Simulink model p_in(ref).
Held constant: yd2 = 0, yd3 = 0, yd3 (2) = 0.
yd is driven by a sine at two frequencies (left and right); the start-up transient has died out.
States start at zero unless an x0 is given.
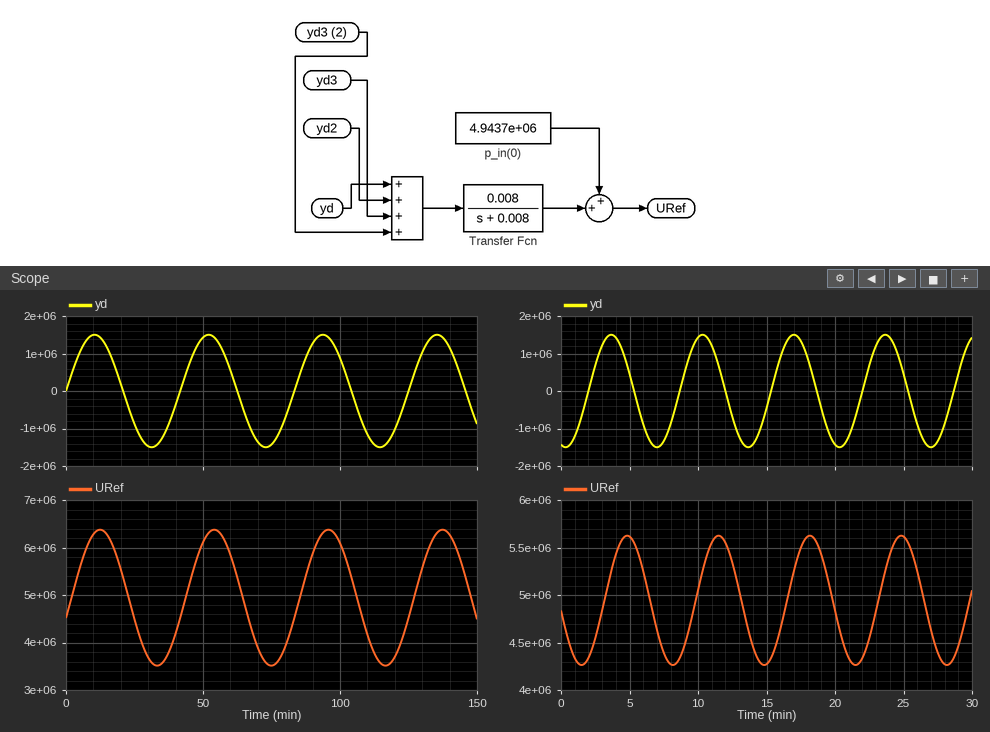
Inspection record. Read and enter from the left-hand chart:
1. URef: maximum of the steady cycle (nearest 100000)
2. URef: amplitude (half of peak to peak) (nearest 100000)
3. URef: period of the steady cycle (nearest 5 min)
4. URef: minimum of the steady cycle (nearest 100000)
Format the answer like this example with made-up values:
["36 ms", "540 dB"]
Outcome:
["6400000", "1400000", "40 min", "3500000"]
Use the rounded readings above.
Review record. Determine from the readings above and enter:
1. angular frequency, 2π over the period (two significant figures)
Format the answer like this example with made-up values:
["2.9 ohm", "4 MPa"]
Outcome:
["0.16 rad/min"]
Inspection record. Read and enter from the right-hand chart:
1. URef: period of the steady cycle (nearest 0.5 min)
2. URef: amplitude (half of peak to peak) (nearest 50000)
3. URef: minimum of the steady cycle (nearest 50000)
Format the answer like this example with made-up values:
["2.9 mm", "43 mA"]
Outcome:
["6.5 min", "700000", "4250000"]
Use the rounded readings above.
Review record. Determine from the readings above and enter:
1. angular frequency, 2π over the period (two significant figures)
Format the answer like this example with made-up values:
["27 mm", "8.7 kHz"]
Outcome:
["0.97 rad/min"]
